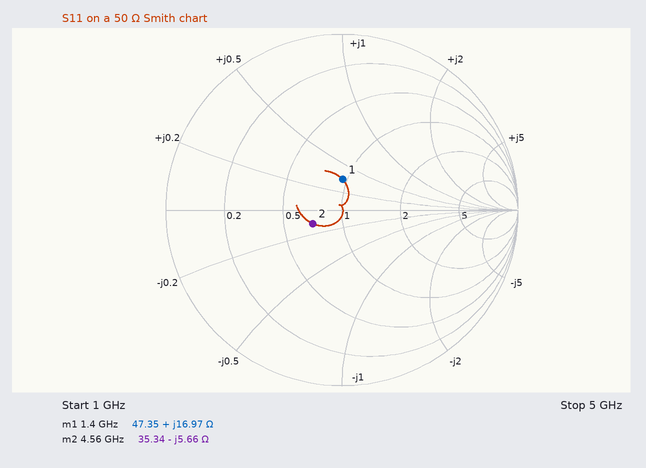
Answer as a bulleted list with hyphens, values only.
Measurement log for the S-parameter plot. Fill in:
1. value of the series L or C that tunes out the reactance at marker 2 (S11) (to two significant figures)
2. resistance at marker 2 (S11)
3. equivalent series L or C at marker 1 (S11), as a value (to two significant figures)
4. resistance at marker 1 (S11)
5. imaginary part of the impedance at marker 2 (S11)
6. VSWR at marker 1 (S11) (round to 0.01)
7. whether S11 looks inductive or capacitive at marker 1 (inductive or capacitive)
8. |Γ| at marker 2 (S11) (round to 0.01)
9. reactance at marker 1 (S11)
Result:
- 200 pH
- 35.34 Ω
- 1.9 nH
- 47.35 Ω
- -5.66 Ω
- 1.42
- inductive
- 0.18
- +16.97 Ω
